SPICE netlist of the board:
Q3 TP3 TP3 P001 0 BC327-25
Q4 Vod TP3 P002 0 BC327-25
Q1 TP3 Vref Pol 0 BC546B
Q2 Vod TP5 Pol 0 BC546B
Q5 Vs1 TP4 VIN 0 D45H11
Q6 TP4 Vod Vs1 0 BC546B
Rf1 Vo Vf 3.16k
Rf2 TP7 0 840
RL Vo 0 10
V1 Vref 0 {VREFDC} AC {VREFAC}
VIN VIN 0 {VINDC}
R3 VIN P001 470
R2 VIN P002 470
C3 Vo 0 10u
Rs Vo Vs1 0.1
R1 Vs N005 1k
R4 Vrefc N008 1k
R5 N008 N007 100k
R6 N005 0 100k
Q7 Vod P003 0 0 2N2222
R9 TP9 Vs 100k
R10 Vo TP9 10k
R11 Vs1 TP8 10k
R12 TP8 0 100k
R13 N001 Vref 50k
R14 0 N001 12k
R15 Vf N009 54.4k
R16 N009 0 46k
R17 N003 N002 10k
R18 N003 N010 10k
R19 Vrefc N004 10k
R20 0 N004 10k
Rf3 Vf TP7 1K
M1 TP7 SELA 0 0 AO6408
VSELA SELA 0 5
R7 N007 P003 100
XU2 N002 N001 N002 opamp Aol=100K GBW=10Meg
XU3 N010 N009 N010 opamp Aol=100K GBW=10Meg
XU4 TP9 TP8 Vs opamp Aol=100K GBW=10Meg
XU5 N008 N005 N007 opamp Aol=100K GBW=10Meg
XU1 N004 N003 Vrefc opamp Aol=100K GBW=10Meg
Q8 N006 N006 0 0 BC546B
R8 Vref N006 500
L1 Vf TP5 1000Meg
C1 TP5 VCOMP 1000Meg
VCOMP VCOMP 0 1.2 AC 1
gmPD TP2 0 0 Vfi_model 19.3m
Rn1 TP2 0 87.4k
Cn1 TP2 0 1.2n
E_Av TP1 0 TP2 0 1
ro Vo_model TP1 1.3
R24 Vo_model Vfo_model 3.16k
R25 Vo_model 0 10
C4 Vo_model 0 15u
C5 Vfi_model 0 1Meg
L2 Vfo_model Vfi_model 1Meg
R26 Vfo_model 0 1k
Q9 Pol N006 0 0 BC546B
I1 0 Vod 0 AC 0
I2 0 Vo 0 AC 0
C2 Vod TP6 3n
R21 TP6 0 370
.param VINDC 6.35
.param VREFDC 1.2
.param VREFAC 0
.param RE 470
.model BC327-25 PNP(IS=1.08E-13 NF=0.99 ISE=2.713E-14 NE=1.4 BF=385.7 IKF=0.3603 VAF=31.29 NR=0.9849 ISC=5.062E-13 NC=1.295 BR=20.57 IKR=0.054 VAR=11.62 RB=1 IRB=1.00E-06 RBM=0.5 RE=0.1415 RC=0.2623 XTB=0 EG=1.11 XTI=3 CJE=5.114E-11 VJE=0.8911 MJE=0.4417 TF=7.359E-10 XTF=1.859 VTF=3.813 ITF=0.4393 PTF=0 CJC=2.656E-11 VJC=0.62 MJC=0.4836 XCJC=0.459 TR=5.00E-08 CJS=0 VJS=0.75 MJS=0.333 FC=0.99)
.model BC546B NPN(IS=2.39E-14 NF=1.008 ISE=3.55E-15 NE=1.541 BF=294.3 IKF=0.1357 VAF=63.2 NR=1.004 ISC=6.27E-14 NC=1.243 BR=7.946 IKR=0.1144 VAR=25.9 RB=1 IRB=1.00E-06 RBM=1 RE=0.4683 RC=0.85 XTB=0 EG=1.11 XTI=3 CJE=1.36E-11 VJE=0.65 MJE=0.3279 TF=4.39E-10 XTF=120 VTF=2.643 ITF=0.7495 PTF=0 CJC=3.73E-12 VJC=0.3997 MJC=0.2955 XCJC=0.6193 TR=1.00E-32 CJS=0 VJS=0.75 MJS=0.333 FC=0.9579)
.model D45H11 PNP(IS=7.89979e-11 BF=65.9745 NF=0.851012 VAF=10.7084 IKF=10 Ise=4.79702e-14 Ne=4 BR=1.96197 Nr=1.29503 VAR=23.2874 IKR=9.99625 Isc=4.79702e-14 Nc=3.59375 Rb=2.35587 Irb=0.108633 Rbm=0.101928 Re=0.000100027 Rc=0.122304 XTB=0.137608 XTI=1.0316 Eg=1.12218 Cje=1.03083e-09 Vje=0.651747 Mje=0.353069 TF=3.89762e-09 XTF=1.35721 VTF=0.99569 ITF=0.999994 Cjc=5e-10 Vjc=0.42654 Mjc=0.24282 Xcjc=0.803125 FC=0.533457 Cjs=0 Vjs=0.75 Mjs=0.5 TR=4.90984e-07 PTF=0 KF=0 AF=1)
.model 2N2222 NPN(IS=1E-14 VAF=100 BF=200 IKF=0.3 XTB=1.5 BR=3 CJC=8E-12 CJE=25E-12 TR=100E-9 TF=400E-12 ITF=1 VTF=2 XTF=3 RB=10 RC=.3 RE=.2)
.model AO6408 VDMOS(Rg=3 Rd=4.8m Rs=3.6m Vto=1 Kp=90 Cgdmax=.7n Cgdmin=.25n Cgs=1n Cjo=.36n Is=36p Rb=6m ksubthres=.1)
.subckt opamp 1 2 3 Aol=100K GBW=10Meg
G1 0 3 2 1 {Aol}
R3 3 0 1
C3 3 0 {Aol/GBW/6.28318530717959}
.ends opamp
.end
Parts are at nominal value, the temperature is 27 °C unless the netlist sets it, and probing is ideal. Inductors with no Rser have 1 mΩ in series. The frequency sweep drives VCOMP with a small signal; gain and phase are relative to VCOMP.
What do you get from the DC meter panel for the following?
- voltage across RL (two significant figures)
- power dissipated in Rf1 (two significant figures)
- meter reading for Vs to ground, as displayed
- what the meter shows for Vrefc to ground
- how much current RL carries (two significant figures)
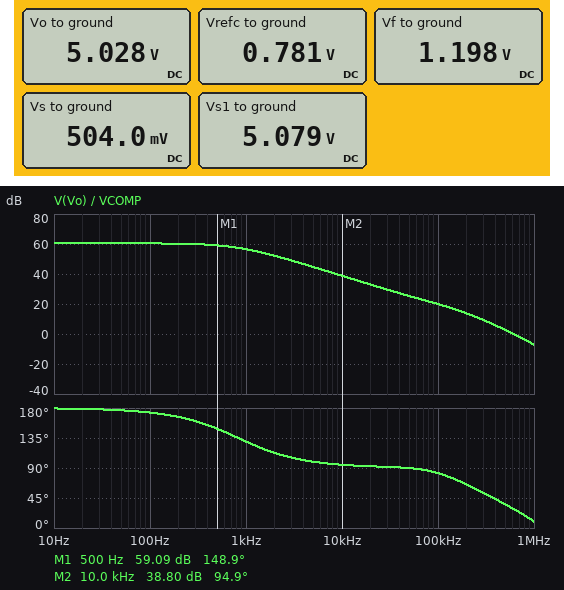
5.0 V
4.6 mW
504.0 mV
0.781 V
500 mA
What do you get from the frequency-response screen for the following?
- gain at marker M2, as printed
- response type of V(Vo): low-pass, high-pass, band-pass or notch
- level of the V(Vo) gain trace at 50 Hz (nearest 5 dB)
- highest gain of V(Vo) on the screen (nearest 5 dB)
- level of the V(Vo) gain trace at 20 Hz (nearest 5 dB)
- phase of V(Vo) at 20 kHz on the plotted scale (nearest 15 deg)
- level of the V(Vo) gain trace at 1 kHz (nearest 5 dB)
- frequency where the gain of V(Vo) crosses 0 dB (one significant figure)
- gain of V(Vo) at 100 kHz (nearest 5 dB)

38.80 dB
low-pass
60 dB
60 dB
60 dB
90 deg
55 dB
600 kHz
20 dB
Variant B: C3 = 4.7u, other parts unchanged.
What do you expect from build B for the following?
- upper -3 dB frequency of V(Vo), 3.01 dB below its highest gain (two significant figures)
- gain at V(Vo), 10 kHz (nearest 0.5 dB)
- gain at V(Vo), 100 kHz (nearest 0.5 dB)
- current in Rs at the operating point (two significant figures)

910 Hz
39.5 dB
21.5 dB
500 mA
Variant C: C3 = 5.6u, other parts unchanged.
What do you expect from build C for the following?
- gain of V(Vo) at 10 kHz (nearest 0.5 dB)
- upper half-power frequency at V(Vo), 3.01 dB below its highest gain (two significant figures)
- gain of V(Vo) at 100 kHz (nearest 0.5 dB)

39.5 dB
890 Hz
21.5 dB
